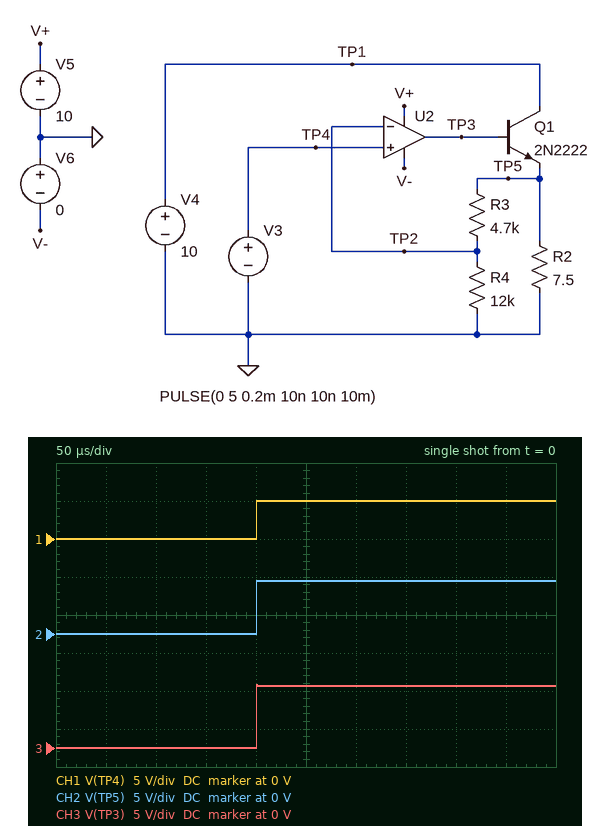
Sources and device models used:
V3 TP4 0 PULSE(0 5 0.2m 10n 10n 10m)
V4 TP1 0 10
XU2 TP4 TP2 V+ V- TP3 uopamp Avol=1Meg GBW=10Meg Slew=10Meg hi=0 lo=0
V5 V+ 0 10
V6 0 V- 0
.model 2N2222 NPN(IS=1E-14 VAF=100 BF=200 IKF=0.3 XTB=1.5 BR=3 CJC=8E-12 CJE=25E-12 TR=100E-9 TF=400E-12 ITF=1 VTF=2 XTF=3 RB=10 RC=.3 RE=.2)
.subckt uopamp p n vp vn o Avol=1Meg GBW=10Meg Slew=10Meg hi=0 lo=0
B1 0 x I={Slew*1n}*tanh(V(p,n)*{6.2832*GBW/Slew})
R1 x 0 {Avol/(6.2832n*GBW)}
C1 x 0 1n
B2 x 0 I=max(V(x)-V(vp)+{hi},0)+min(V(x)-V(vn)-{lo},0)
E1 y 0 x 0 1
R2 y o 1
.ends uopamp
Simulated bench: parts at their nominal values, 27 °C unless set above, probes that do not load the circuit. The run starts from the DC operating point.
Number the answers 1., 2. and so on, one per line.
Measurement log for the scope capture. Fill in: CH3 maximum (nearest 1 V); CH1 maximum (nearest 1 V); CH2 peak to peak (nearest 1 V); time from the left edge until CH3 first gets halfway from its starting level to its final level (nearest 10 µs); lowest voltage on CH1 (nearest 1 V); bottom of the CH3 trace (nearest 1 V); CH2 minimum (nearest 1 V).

1. 8 V
2. 5 V
3. 7 V
4. 200 µs
5. 0 V
6. 0 V
7. 0 V
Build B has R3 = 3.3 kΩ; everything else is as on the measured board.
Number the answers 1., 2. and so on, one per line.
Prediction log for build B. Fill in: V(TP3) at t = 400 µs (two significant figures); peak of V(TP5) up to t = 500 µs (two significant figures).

1. 7.6 V
2. 6.4 V
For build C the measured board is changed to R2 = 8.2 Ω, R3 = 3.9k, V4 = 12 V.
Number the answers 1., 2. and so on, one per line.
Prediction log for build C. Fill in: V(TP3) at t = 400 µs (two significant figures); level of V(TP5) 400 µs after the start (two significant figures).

1. 7.8 V
2. 6.6 V
